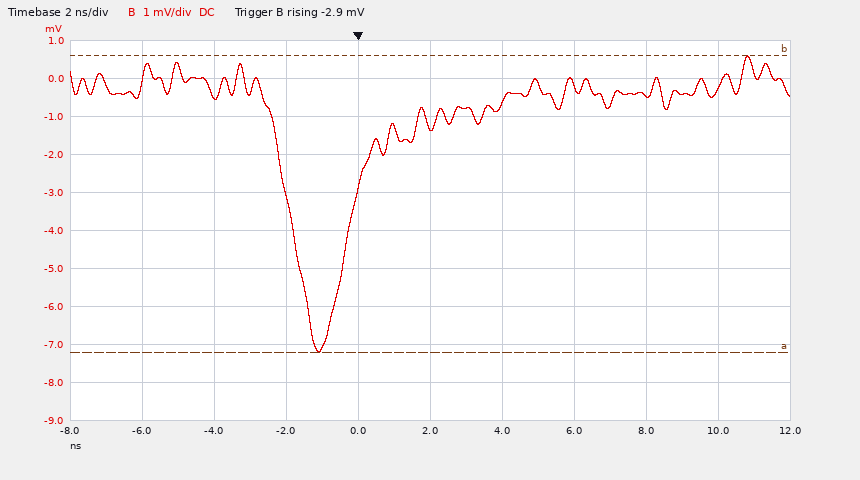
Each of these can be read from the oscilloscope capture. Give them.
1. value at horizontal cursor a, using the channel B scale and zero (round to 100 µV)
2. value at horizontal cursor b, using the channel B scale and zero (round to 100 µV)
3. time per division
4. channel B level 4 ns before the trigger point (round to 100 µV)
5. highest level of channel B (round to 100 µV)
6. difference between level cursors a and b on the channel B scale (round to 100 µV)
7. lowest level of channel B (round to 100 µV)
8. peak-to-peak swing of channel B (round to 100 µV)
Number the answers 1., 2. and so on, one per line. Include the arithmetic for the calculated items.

1. -7.2 mV
2. 600 µV
3. 2 ns
4. -500 µV
5. 600 µV
6. 7.8 mV
7. -7.2 mV
8. 600 µV − (-7.2 mV) = 7.8 mV
